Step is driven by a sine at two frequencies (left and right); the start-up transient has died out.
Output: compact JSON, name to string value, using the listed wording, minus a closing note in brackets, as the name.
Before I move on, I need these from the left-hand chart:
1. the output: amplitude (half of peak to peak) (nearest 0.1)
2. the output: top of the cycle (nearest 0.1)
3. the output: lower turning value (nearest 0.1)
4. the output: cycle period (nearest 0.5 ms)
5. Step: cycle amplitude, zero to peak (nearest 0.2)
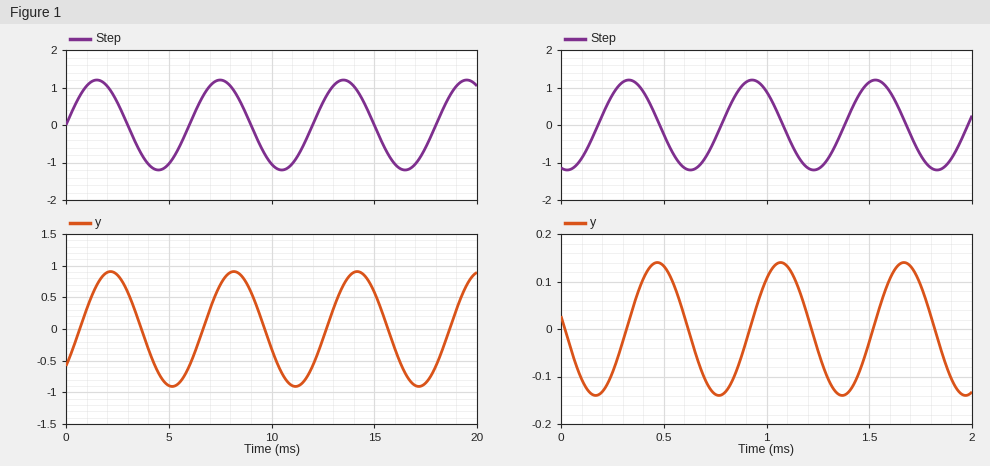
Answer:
{"the output: amplitude (half of peak to peak)": "0.9", "the output: top of the cycle": "0.9", "the output: lower turning value": "-0.9", "the output: cycle period": "6.0 ms", "Step: cycle amplitude, zero to peak": "1.2"}
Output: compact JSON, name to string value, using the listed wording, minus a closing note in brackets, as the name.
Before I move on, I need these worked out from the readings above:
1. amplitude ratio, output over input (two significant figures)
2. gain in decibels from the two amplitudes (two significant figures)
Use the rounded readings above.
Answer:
{"amplitude ratio, output over input": "0.75", "gain in decibels from the two amplitudes": "-2.5 dB"}
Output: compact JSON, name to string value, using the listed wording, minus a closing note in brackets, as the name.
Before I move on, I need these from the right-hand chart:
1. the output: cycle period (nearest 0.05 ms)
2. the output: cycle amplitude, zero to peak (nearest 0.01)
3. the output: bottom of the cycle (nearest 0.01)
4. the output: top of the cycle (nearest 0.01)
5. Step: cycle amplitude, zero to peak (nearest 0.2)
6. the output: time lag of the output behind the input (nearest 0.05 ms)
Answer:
{"the output: cycle period": "0.60 ms", "the output: cycle amplitude, zero to peak": "0.14", "the output: bottom of the cycle": "-0.14", "the output: top of the cycle": "0.14", "Step: cycle amplitude, zero to peak": "1.2", "the output: time lag of the output behind the input": "0.15 ms"}
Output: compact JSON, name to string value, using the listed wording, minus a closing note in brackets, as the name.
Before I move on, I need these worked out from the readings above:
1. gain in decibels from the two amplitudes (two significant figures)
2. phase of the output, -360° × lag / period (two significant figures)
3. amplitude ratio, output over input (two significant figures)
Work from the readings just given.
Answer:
{"gain in decibels from the two amplitudes": "-19 dB", "phase of the output, -360° × lag / period": "-90°", "amplitude ratio, output over input": "0.12"}
